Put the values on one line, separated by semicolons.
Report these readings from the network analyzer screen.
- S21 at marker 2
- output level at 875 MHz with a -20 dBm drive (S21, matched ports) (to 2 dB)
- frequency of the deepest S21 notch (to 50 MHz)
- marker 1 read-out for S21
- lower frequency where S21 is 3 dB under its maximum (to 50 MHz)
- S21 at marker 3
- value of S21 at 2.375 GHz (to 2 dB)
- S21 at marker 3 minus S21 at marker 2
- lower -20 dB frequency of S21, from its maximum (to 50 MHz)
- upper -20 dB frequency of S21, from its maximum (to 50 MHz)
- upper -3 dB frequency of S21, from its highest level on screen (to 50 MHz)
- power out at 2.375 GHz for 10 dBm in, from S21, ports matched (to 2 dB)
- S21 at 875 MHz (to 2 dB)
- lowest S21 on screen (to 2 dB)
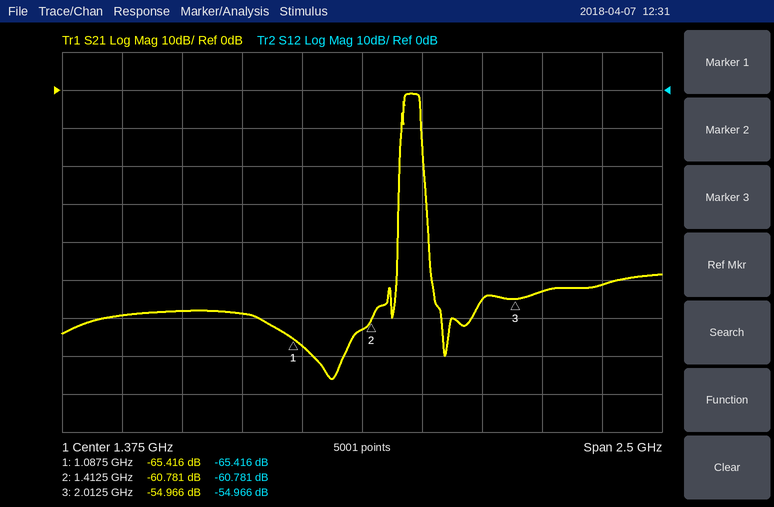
-60.781 dB; -78 dBm; 1.25 GHz; -65.416 dB; 1.55 GHz; -54.966 dB; -52 dB; 5.815 dB; 1.55 GHz; 1.65 GHz; 1.60 GHz; -42 dBm; -58 dB; -76 dB
